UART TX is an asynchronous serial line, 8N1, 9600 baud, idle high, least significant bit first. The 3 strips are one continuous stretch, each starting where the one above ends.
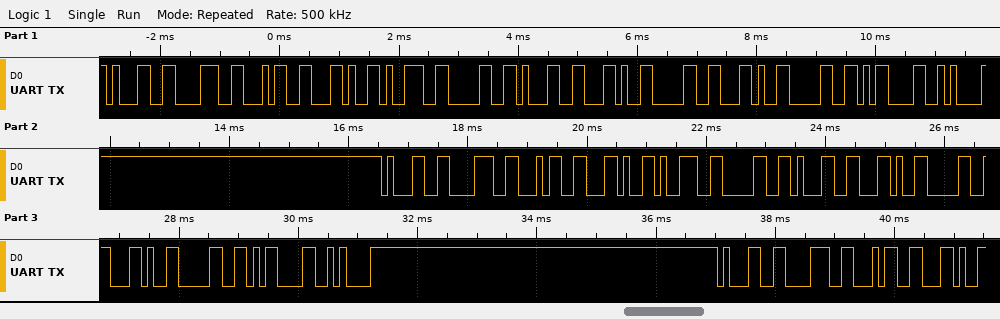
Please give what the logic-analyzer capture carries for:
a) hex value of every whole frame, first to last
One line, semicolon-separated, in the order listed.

31 38 34 2C 39 30 31 2C 30 2C 30 0D 0A 31 38 34 2C 39 30 31 2C 30 2C 30 0D 0A 31 38 34 2C
